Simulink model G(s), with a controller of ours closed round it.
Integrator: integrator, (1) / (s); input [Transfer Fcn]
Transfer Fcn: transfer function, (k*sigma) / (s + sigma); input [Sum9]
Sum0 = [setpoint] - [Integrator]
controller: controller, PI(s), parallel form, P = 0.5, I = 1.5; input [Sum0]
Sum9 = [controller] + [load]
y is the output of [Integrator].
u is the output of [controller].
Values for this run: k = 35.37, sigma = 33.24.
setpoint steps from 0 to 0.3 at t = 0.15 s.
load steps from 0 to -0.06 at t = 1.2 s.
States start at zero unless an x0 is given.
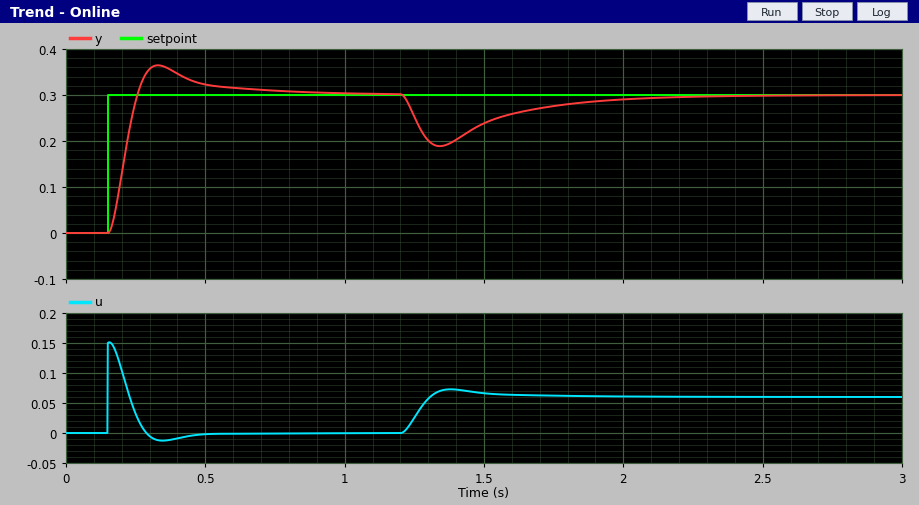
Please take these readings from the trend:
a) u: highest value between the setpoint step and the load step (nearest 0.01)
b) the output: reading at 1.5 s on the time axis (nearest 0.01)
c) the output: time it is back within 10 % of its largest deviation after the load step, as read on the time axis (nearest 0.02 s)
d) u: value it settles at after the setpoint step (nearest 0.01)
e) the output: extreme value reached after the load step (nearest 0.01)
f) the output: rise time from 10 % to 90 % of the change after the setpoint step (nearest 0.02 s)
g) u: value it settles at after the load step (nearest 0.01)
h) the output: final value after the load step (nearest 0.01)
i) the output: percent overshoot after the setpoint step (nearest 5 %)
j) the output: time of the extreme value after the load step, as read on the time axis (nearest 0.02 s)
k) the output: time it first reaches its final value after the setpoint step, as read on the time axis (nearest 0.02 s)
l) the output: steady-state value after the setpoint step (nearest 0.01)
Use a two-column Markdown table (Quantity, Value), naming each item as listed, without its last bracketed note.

| Quantity | Value |
|---|---|
| u: highest value between the setpoint step and the load step | 0.15 |
| the output: reading at 1.5 s on the time axis | 0.24 |
| the output: time it is back within 10 % of its largest deviation after the load step, as read on the time axis | 1.96 s |
| u: value it settles at after the setpoint step | 0.00 |
| the output: extreme value reached after the load step | 0.19 |
| the output: rise time from 10 % to 90 % of the change after the setpoint step | 0.08 s |
| u: value it settles at after the load step | 0.06 |
| the output: final value after the load step | 0.30 |
| the output: percent overshoot after the setpoint step | 20 % |
| the output: time of the extreme value after the load step, as read on the time axis | 1.34 s |
| the output: time it first reaches its final value after the setpoint step, as read on the time axis | 0.26 s |
| the output: steady-state value after the setpoint step | 0.30 |
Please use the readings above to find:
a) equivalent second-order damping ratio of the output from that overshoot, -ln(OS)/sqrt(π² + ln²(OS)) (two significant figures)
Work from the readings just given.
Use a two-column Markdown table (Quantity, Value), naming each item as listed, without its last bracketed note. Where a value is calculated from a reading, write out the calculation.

| Quantity | Value |
|---|---|
| equivalent second-order damping ratio of the output from that overshoot, -ln(OS)/sqrt(π² + ln²(OS)) | ln(0.2) = -1.609; 1.609 / sqrt(9.870 + 2.590) = 0.46 |
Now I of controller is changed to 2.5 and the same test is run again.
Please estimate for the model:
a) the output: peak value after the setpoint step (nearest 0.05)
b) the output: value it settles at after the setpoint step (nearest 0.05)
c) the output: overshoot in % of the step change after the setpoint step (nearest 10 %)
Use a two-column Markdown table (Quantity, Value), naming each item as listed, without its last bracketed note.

| Quantity | Value |
|---|---|
| the output: peak value after the setpoint step | 0.40 |
| the output: value it settles at after the setpoint step | 0.30 |
| the output: overshoot in % of the step change after the setpoint step | 30 % |
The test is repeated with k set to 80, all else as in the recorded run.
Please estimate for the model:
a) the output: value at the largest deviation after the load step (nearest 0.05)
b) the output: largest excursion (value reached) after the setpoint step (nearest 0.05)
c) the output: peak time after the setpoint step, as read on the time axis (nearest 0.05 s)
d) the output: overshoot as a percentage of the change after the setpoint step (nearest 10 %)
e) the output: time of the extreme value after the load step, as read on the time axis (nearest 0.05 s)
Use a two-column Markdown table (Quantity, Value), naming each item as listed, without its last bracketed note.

| Quantity | Value |
|---|---|
| the output: value at the largest deviation after the load step | 0.15 |
| the output: largest excursion (value reached) after the setpoint step | 0.40 |
| the output: peak time after the setpoint step, as read on the time axis | 0.25 s |
| the output: overshoot as a percentage of the change after the setpoint step | 30 % |
| the output: time of the extreme value after the load step, as read on the time axis | 1.30 s |
